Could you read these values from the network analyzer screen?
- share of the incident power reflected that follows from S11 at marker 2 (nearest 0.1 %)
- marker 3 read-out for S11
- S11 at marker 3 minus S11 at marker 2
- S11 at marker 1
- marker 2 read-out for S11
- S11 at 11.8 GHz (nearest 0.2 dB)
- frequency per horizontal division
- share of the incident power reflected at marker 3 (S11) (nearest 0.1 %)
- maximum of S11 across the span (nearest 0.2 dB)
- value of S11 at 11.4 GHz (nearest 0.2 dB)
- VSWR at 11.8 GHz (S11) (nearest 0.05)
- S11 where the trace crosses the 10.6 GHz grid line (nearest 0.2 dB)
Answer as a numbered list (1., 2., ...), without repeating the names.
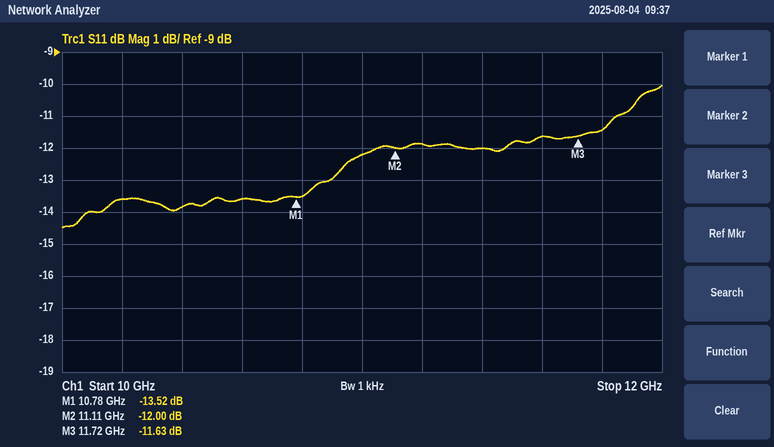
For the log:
1. 6.3 %
2. -11.63 dB
3. 0.37 dB
4. -13.52 dB
5. -12.00 dB
6. -11.4 dB
7. 200 MHz
8. 6.9 %
9. -10.0 dB
10. -12.0 dB
11. 1.75
12. -13.6 dB
